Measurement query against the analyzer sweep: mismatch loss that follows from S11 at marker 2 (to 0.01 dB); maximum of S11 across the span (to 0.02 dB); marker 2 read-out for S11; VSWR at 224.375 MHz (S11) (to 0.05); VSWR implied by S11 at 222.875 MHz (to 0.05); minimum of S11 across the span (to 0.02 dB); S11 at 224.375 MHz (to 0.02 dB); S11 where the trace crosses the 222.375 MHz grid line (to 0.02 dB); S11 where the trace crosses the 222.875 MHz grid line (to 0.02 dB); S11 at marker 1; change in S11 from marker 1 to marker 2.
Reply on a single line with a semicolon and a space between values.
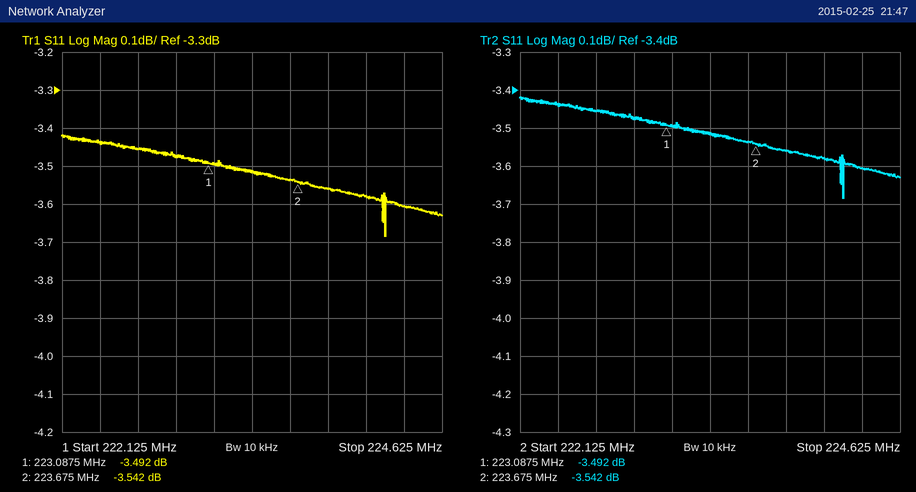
2.54 dB; -3.42 dB; -3.542 dB; 4.90; 5.05; -3.68 dB; -3.60 dB; -3.44 dB; -3.48 dB; -3.492 dB; -0.050 dB
